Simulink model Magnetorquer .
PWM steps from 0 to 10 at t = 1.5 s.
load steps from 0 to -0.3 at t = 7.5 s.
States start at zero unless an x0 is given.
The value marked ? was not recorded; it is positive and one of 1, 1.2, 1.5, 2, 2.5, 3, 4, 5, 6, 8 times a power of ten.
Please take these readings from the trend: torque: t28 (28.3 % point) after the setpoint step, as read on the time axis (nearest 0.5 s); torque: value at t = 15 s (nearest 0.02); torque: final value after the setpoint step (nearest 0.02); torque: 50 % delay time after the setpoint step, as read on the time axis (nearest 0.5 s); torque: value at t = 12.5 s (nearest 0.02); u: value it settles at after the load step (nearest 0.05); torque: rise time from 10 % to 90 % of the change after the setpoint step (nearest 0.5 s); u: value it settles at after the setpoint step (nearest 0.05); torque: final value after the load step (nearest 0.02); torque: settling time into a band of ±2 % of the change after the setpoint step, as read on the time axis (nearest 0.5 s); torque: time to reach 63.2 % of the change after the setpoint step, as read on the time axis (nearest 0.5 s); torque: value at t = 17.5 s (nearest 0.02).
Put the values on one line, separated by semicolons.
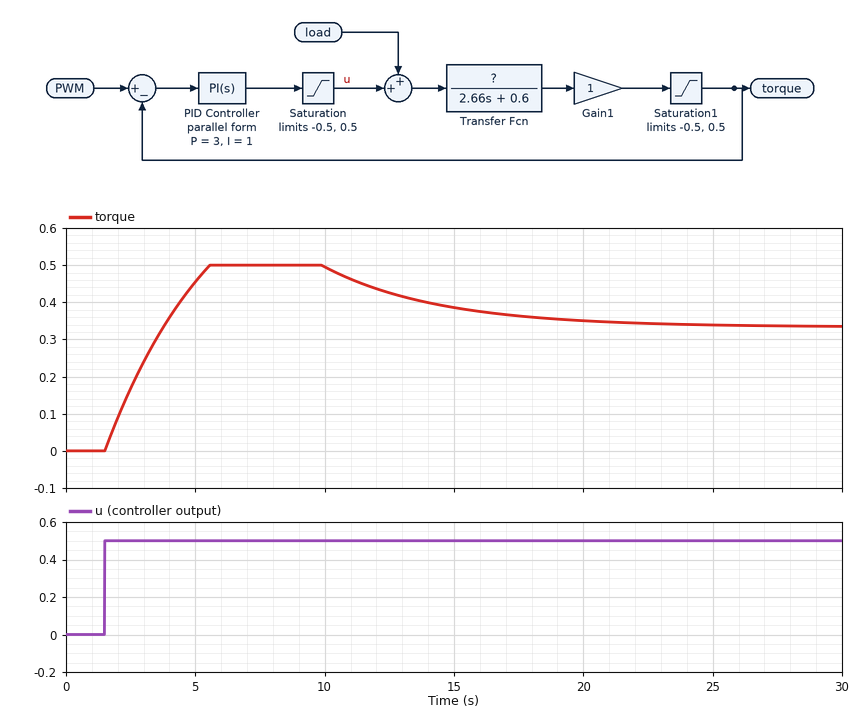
2.5 s; 0.38; 0.50; 3.0 s; 0.42; 0.50; 3.0 s; 0.50; 0.34; 5.5 s; 3.5 s; 0.36
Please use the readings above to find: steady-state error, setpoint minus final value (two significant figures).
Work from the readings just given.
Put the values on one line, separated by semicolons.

9.5
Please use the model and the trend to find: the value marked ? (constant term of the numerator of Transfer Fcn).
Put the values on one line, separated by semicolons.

1
